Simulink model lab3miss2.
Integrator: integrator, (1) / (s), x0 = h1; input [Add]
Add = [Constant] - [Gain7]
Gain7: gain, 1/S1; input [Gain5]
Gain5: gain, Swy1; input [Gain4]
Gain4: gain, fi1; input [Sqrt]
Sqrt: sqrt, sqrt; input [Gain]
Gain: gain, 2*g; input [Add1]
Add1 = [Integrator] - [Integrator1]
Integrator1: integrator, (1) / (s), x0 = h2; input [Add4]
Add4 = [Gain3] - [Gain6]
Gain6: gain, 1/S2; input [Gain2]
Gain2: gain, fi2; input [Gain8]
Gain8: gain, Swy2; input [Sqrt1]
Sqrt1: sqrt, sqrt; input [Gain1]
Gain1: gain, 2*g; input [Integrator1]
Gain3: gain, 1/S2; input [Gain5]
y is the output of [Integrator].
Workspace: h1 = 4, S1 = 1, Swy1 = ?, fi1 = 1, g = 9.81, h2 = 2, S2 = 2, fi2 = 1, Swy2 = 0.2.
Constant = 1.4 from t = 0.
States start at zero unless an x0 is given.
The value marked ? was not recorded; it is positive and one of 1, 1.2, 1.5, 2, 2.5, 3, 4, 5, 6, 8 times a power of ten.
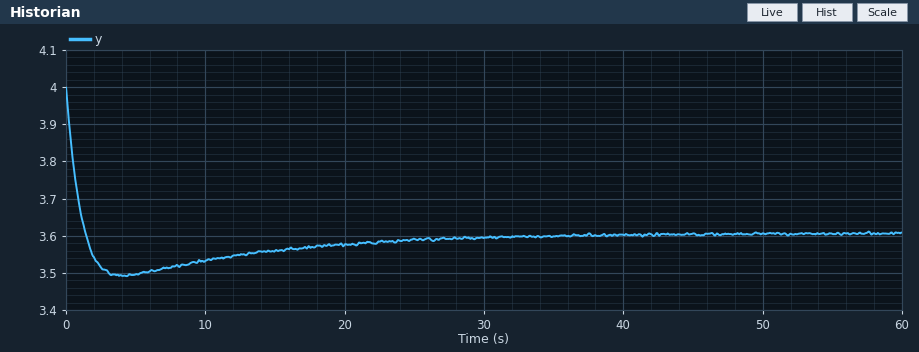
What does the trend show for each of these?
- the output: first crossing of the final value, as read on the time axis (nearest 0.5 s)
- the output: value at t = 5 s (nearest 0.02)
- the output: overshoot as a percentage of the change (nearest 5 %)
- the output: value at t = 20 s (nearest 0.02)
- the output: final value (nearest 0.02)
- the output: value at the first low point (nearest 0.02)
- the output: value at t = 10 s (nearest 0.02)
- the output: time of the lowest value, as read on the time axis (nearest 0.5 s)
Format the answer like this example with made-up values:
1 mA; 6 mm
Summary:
1.5 s; 3.50; 30 %; 3.58; 3.60; 3.50; 3.54; 4.0 s
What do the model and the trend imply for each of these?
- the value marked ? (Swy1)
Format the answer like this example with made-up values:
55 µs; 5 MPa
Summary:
0.3
